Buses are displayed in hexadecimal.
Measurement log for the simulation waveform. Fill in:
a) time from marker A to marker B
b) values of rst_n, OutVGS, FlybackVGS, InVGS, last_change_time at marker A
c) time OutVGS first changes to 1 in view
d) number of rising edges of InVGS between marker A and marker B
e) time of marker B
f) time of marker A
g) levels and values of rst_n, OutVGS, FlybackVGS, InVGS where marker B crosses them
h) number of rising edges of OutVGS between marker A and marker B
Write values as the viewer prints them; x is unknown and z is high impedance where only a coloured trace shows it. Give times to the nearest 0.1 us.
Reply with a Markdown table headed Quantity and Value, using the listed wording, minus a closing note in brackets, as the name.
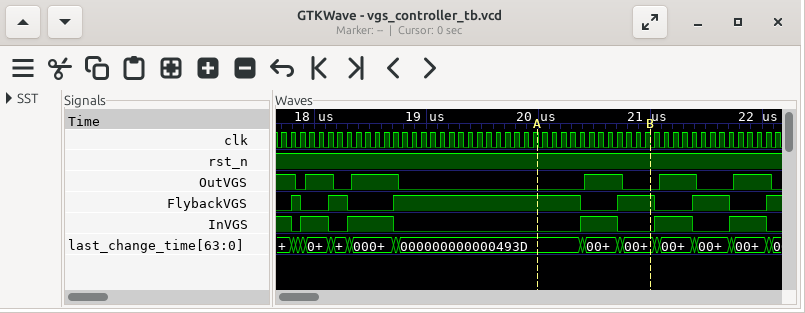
| Quantity | Value |
|---|---|
| time from marker A to marker B | 1 us |
| values of rst_n, OutVGS, FlybackVGS, InVGS, last_change_time at marker A | rst_n=1, OutVGS=0, FlybackVGS=1, InVGS=0, last_change_time=000000000000493D |
| time OutVGS first changes to 1 in view | 17.9 us |
| number of rising edges of InVGS between marker A and marker B | 1 |
| time of marker B | 21 us |
| time of marker A | 20 us |
| levels and values of rst_n, OutVGS, FlybackVGS, InVGS where marker B crosses them | rst_n=1, OutVGS=0, FlybackVGS=1, InVGS=0 |
| number of rising edges of OutVGS between marker A and marker B | 1 |
